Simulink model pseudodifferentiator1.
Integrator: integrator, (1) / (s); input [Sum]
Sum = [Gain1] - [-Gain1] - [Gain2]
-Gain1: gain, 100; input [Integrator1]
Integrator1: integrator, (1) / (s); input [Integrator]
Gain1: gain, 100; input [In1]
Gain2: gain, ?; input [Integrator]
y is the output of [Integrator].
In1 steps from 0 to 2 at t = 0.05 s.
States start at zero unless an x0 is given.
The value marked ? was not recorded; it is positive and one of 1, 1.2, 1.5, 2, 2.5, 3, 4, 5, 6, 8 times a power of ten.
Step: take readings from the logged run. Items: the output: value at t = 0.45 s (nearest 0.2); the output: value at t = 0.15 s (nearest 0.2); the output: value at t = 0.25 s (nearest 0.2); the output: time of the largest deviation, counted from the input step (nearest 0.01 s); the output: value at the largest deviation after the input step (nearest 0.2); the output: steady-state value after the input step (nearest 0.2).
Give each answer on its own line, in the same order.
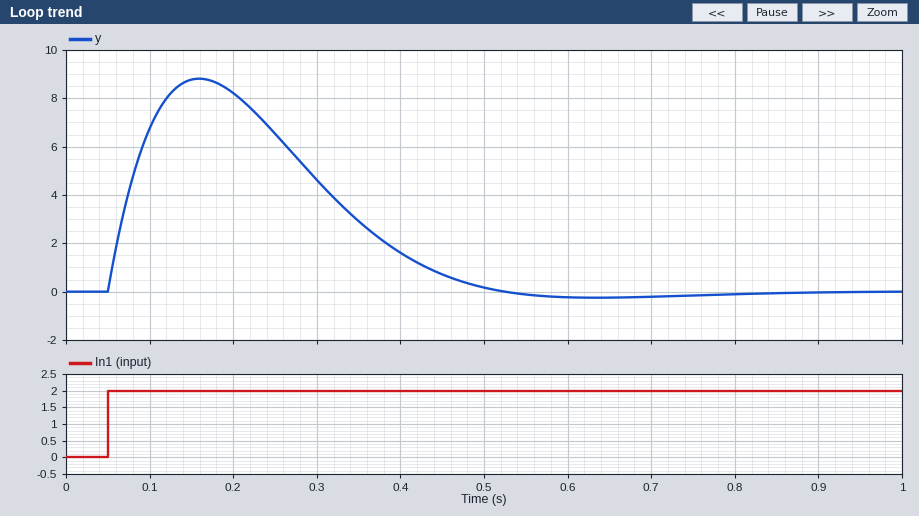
0.8
8.8
6.6
0.11 s
8.8
0.0
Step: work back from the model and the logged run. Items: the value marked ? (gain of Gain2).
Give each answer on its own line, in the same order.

15
